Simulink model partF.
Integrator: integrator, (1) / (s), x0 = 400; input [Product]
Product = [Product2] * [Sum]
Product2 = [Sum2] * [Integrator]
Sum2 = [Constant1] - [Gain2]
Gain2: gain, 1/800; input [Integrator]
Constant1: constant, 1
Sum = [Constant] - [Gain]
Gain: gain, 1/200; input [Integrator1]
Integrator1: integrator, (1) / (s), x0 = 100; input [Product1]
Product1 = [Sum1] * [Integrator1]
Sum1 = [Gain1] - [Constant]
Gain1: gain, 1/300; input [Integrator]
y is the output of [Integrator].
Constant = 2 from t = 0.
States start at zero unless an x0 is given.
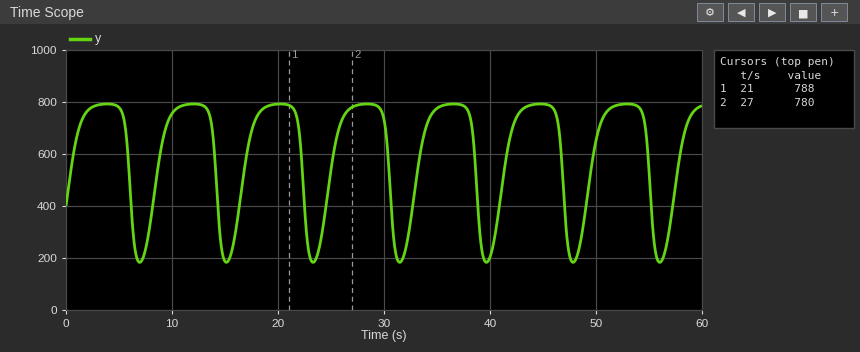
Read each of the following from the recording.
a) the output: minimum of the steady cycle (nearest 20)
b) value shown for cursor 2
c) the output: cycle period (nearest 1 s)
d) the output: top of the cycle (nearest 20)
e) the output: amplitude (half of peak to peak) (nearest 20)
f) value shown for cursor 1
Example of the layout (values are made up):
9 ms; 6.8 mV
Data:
180; 780; 8 s; 800; 300; 788
